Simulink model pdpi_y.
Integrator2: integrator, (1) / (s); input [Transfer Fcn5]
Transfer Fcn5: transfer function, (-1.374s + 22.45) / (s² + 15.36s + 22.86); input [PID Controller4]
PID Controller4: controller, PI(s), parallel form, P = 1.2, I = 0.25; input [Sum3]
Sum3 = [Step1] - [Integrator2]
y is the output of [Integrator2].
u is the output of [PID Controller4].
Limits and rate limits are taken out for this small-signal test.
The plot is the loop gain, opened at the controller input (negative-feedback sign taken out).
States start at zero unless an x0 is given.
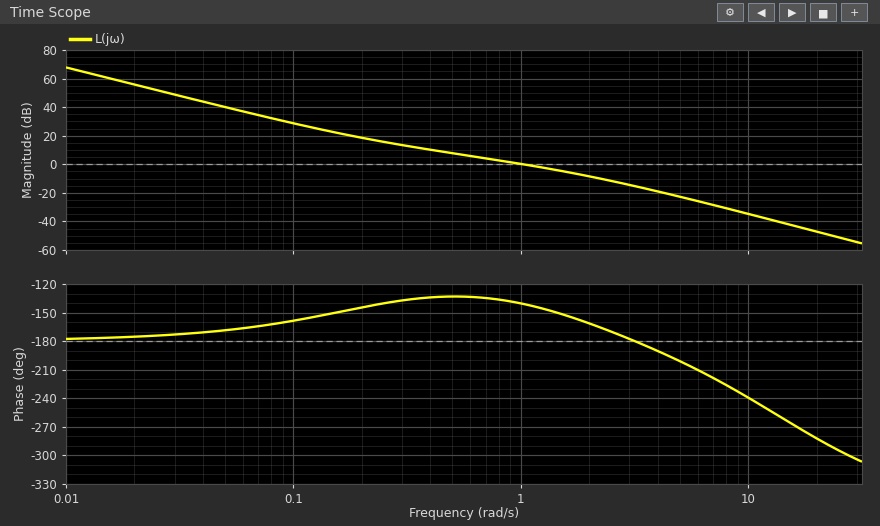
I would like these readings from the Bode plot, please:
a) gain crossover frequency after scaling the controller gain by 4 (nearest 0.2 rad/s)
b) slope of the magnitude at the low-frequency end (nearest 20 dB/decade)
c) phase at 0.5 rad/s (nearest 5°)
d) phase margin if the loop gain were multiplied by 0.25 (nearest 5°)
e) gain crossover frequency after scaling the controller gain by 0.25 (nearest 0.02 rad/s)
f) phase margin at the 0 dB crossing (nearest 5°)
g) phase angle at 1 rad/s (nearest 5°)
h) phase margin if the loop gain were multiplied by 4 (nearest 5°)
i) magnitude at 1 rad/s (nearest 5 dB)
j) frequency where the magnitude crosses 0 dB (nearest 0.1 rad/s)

2.6 rad/s
-40 dB/decade
-135°
45°
0.34 rad/s
40°
-140°
10°
0 dB
1.0 rad/s
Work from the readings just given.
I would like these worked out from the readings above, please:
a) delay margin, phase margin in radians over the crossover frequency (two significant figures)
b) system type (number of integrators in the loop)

0.70 s
2
